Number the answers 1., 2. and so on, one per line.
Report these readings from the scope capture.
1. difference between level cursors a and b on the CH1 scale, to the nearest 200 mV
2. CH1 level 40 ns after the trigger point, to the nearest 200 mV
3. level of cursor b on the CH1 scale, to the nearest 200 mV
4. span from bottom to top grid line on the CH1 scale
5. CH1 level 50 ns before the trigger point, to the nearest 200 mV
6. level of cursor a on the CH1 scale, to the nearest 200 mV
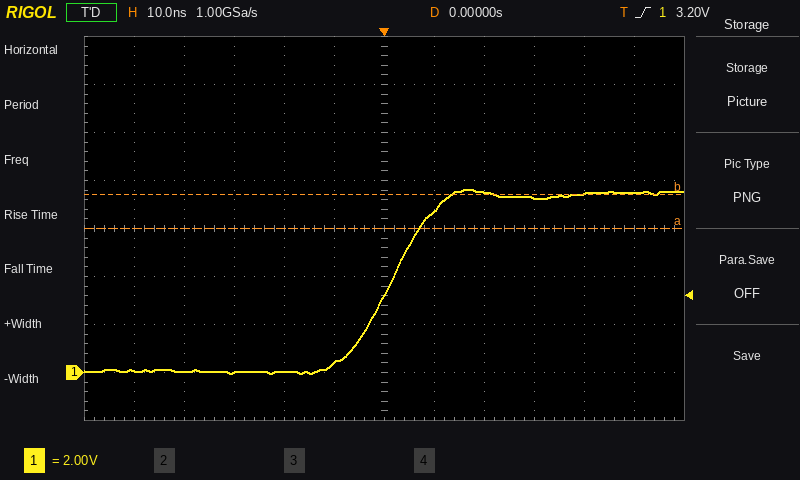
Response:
1. 1.4 V
2. 7.4 V
3. 7.4 V
4. 16 V
5. 0.0 V
6. 6.0 V
